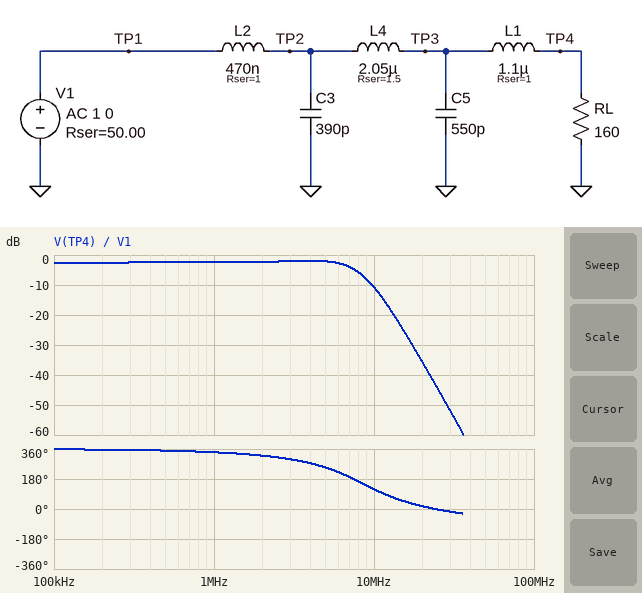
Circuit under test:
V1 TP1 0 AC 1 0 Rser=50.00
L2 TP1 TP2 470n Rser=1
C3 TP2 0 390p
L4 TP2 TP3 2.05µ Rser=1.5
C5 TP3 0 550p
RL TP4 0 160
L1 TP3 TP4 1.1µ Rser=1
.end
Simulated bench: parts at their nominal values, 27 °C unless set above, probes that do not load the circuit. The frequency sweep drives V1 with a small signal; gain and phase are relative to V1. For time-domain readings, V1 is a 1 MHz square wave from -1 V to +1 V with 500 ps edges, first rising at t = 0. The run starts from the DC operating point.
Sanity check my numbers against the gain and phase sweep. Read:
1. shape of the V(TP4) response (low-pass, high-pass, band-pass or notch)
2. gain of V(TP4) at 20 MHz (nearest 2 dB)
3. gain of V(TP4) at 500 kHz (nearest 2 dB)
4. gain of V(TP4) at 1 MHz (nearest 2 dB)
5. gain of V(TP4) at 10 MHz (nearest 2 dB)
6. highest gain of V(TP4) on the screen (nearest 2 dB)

low-pass
-36 dB
-2 dB
-2 dB
-10 dB
-2 dB
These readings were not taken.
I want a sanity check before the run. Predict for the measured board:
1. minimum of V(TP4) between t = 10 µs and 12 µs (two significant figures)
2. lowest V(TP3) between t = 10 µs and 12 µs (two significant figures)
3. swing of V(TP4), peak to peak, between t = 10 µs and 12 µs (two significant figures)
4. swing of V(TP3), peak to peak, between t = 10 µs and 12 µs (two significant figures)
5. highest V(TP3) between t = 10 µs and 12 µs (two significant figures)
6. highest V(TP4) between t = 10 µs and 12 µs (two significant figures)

-960 mV
-980 mV
1.9 V
2.0 V
980 mV
960 mV
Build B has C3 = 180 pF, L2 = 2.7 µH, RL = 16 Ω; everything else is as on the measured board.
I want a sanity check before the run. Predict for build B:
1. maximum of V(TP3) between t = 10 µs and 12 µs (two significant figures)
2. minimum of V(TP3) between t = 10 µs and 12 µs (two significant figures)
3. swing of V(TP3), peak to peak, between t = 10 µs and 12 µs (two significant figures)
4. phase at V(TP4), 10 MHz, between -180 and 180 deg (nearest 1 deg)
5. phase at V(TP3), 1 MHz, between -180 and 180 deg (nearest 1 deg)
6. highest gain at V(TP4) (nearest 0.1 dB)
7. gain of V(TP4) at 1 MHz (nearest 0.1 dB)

610 mV
-610 mV
1.2 V
110 deg
-9 deg
-12.2 dB
-13.6 dB
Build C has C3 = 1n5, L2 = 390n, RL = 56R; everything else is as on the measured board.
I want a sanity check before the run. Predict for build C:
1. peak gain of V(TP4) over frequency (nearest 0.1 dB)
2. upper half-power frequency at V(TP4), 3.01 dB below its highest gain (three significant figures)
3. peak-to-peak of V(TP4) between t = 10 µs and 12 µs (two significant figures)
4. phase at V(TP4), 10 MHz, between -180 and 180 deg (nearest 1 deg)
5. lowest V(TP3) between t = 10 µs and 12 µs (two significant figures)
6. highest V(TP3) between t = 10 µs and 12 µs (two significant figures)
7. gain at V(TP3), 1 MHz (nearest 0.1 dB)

-5.8 dB
4.77 MHz
1.1 V
49 deg
-570 mV
570 mV
-5.7 dB
